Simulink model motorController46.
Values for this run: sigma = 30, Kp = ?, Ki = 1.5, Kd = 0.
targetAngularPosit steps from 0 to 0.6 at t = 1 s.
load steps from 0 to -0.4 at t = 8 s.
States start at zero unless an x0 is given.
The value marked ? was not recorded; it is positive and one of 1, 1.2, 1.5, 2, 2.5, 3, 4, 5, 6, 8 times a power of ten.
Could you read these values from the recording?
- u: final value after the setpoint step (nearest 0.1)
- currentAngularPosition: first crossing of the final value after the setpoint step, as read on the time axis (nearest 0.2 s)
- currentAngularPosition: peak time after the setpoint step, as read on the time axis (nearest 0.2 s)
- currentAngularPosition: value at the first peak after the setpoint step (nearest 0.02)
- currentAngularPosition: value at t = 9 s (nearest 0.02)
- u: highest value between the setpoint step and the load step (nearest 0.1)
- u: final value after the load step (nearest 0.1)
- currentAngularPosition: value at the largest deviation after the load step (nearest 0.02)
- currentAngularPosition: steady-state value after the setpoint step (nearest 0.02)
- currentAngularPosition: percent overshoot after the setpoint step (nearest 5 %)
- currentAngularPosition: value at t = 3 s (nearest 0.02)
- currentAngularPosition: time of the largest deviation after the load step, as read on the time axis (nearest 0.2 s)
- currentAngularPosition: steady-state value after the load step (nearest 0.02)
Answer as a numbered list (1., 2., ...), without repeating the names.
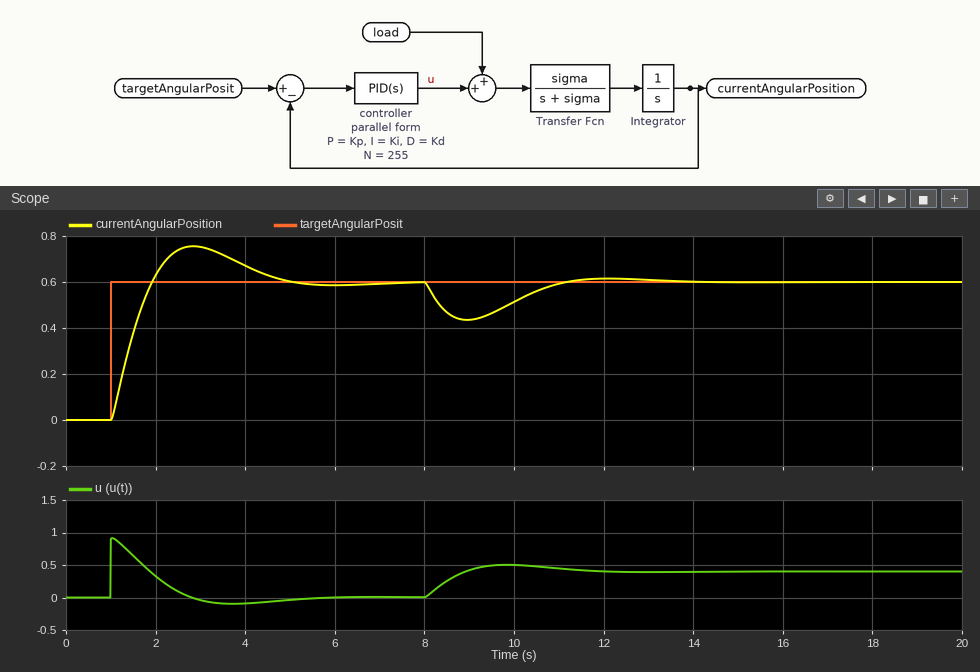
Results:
1. 0.0
2. 2.0 s
3. 2.8 s
4. 0.76
5. 0.44
6. 0.9
7. 0.4
8. 0.44
9. 0.60
10. 25 %
11. 0.76
12. 9.0 s
13. 0.60
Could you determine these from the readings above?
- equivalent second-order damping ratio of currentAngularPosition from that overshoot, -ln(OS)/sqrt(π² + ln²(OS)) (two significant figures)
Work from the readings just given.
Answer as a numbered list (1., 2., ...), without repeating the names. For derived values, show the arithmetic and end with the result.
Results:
1. ln(0.25) = -1.386; 1.386 / sqrt(9.870 + 1.922) = 0.40
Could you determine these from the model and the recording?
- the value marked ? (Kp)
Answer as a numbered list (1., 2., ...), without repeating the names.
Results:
1. 1.5
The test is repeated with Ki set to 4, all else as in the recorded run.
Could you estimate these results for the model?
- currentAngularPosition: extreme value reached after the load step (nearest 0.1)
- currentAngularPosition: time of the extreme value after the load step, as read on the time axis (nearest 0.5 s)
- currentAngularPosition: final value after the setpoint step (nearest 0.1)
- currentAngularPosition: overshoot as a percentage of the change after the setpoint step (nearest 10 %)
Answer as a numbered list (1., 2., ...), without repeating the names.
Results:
1. 0.5
2. 8.5 s
3. 0.6
4. 40 %
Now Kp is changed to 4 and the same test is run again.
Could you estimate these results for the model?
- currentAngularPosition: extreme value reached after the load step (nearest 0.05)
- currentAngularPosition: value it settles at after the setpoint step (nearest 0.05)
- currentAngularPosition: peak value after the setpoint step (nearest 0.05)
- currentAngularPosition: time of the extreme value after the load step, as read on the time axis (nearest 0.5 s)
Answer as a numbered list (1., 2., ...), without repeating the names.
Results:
1. 0.50
2. 0.60
3. 0.65
4. 8.5 s
